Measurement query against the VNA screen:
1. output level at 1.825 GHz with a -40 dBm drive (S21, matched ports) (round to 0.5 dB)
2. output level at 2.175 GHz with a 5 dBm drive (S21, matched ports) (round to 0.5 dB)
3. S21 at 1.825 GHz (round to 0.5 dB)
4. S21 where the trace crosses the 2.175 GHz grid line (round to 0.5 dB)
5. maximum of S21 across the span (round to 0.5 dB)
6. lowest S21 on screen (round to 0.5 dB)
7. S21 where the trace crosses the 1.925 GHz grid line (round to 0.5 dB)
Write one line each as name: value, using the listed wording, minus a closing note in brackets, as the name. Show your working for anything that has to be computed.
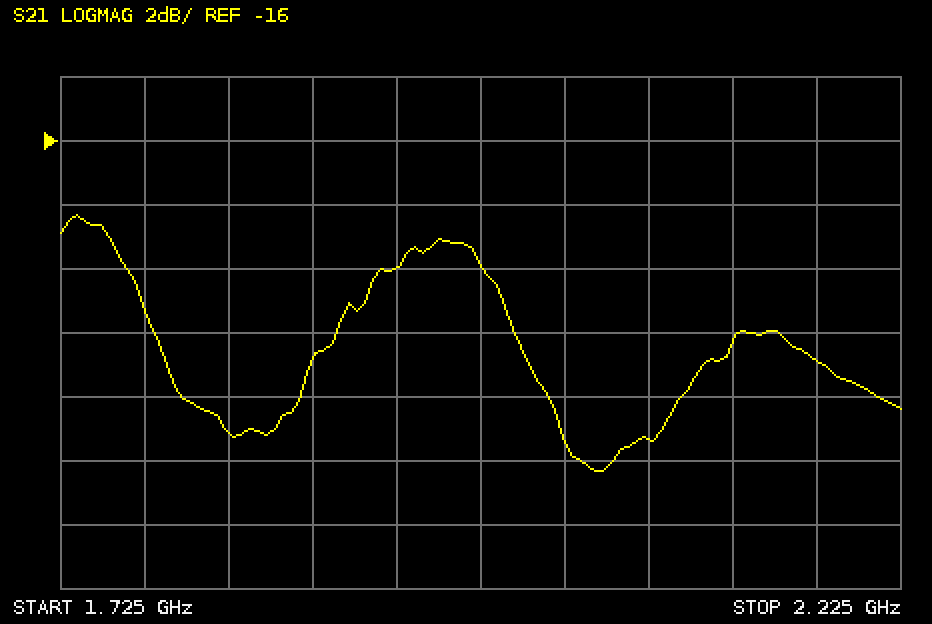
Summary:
output level at 1.825 GHz with a -40 dBm drive (S21, matched ports): -40 dBm + (-25.0 dB) = -65.0 dBm
output level at 2.175 GHz with a 5 dBm drive (S21, matched ports): 5 dBm + (-23.0 dB) = -18.0 dBm
S21 at 1.825 GHz: -25.0 dB
S21 where the trace crosses the 2.175 GHz grid line: -23.0 dB
maximum of S21 across the span: -18.5 dB
lowest S21 on screen: -26.5 dB
S21 where the trace crosses the 1.925 GHz grid line: -20.0 dB
